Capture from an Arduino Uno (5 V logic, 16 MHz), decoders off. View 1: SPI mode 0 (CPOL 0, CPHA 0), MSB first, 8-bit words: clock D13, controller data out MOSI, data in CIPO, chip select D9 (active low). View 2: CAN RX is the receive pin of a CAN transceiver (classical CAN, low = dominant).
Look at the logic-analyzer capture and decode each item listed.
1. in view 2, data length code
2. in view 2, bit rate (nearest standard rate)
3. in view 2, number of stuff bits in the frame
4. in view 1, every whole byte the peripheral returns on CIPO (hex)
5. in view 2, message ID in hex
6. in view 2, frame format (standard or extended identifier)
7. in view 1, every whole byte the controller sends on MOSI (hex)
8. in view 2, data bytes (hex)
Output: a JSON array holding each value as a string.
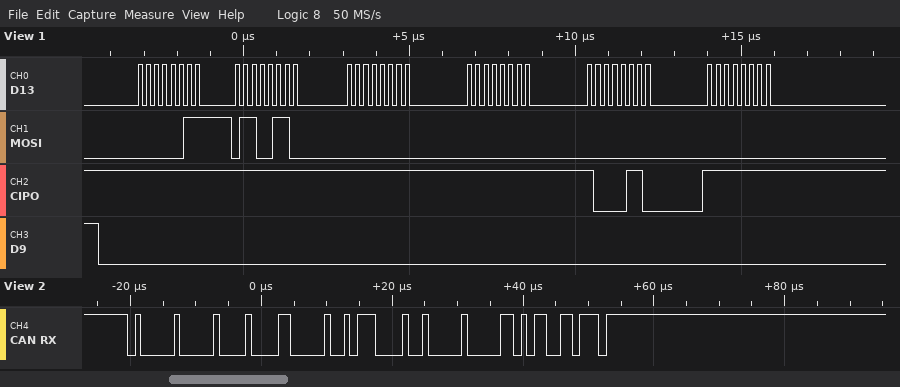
["4", "1000 kbit/s", "5", "FF FF FF FF 86 FF", "0x400", "standard", "03 66 00 00 00 00", "30 17 09 00"]
